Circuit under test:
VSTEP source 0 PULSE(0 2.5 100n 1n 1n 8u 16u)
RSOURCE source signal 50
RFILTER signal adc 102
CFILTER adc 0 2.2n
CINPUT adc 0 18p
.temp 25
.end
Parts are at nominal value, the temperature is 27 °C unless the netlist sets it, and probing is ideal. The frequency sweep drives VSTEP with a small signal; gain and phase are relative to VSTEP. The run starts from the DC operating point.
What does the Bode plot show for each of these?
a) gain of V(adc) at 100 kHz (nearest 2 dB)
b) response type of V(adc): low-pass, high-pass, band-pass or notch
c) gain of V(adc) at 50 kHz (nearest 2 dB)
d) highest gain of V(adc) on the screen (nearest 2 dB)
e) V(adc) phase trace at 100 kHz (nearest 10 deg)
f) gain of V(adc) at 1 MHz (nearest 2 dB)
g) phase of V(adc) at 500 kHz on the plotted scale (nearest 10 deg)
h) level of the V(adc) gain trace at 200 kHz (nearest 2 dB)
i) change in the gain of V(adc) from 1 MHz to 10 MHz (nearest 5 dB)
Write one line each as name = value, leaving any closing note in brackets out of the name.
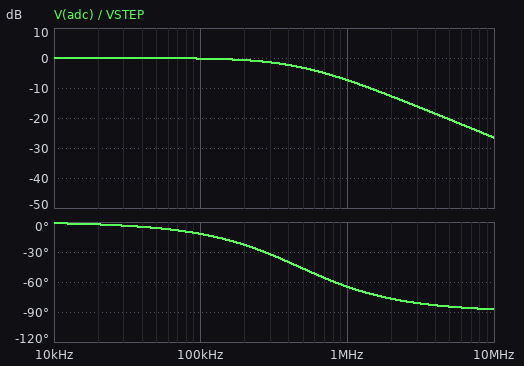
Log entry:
gain of V(adc) at 100 kHz = 0 dB
response type of V(adc): low-pass, high-pass, band-pass or notch = low-pass
gain of V(adc) at 50 kHz = 0 dB
highest gain of V(adc) on the screen = 0 dB
V(adc) phase trace at 100 kHz = -10 deg
gain of V(adc) at 1 MHz = -8 dB
phase of V(adc) at 500 kHz on the plotted scale = -50 deg
level of the V(adc) gain trace at 200 kHz = 0 dB
change in the gain of V(adc) from 1 MHz to 10 MHz = -20 dB
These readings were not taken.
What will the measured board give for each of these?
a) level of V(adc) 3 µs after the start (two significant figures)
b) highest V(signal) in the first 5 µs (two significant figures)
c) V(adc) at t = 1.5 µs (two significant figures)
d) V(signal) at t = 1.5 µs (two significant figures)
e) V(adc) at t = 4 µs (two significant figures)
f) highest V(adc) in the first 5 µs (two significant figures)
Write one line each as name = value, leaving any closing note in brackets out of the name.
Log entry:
level of V(adc) 3 µs after the start = 2.5 V
highest V(signal) in the first 5 µs = 2.5 V
V(adc) at t = 1.5 µs = 2.5 V
V(signal) at t = 1.5 µs = 2.5 V
V(adc) at t = 4 µs = 2.5 V
highest V(adc) in the first 5 µs = 2.5 V
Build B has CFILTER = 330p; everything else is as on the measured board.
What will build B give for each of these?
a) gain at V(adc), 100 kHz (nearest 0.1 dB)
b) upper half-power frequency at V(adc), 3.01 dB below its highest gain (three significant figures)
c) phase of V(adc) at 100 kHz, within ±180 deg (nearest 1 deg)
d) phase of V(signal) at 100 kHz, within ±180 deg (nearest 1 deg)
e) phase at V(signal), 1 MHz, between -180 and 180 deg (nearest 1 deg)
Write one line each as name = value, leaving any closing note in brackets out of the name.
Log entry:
gain at V(adc), 100 kHz = 0 dB
upper half-power frequency at V(adc), 3.01 dB below its highest gain = 3.01 MHz
phase of V(adc) at 100 kHz, within ±180 deg = -2 deg
phase of V(signal) at 100 kHz, within ±180 deg = -1 deg
phase at V(signal), 1 MHz, between -180 and 180 deg = -6 deg
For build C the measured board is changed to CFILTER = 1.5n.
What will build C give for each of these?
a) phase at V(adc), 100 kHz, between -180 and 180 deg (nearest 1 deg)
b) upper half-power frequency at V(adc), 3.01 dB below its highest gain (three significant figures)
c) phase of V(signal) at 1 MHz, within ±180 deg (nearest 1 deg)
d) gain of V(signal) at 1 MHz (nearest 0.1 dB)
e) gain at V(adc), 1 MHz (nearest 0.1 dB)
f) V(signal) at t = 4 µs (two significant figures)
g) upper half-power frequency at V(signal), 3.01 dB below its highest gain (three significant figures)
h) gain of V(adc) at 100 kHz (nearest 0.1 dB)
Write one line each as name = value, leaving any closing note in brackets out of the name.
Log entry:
phase at V(adc), 100 kHz, between -180 and 180 deg = -8 deg
upper half-power frequency at V(adc), 3.01 dB below its highest gain = 690 kHz
phase of V(signal) at 1 MHz, within ±180 deg = -11 deg
gain of V(signal) at 1 MHz = -2.0 dB
gain at V(adc), 1 MHz = -4.9 dB
V(signal) at t = 4 µs = 2.5 V
upper half-power frequency at V(signal), 3.01 dB below its highest gain = 2.19 MHz
gain of V(adc) at 100 kHz = -0.1 dB
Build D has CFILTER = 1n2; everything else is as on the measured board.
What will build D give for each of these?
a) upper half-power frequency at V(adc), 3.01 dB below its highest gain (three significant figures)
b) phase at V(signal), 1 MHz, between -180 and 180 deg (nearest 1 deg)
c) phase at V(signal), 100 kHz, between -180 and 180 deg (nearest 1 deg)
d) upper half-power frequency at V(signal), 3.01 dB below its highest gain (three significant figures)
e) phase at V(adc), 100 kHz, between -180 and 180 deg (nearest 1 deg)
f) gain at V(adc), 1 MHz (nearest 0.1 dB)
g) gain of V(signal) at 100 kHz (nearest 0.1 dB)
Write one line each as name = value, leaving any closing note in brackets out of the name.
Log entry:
upper half-power frequency at V(adc), 3.01 dB below its highest gain = 860 kHz
phase at V(signal), 1 MHz, between -180 and 180 deg = -11 deg
phase at V(signal), 100 kHz, between -180 and 180 deg = -2 deg
upper half-power frequency at V(signal), 3.01 dB below its highest gain = 2.73 MHz
phase at V(adc), 100 kHz, between -180 and 180 deg = -7 deg
gain at V(adc), 1 MHz = -3.7 dB
gain of V(signal) at 100 kHz = 0 dB
